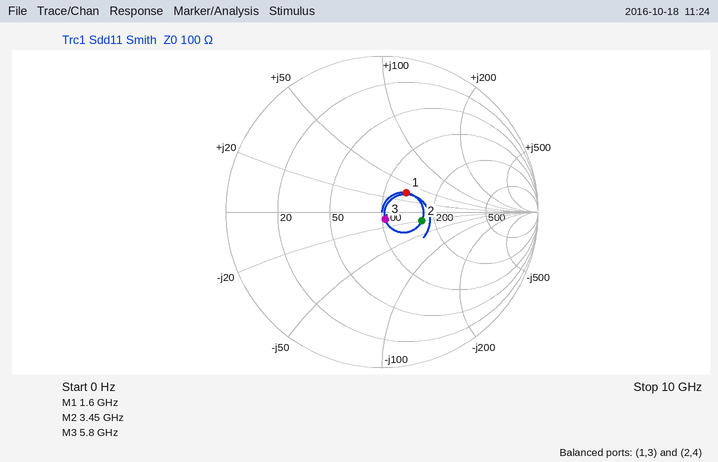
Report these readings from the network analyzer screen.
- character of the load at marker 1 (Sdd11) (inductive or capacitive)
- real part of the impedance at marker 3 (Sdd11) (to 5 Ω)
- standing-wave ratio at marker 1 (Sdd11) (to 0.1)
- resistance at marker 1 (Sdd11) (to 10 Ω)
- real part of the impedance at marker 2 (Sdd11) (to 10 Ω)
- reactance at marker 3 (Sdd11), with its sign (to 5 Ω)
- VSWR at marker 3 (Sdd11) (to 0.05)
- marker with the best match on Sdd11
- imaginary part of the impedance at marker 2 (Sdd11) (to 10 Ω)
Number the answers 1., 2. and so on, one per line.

1. inductive
2. 105 Ω
3. 1.5
4. 130 Ω
5. 170 Ω
6. -10 Ω
7. 1.10
8. marker 3
9. -20 Ω
